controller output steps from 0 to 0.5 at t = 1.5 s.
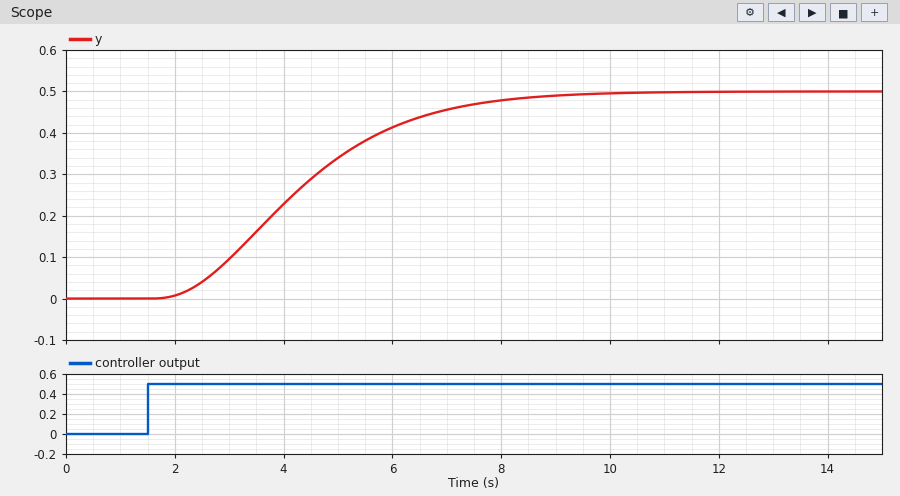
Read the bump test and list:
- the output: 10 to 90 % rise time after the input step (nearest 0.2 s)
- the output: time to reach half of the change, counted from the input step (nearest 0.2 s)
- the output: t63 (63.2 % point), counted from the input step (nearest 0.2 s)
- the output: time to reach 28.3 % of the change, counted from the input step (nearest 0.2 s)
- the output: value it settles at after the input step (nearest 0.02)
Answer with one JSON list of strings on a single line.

["4.2 s", "2.6 s", "3.2 s", "1.8 s", "0.50"]
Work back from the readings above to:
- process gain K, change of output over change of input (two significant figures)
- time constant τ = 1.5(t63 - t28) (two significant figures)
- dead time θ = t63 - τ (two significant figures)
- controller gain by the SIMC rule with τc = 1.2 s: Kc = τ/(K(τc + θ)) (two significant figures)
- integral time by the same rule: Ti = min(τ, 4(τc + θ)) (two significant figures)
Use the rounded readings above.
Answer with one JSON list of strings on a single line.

["1.0", "2.1 s", "1.1 s", "0.91", "2.1 s"]
